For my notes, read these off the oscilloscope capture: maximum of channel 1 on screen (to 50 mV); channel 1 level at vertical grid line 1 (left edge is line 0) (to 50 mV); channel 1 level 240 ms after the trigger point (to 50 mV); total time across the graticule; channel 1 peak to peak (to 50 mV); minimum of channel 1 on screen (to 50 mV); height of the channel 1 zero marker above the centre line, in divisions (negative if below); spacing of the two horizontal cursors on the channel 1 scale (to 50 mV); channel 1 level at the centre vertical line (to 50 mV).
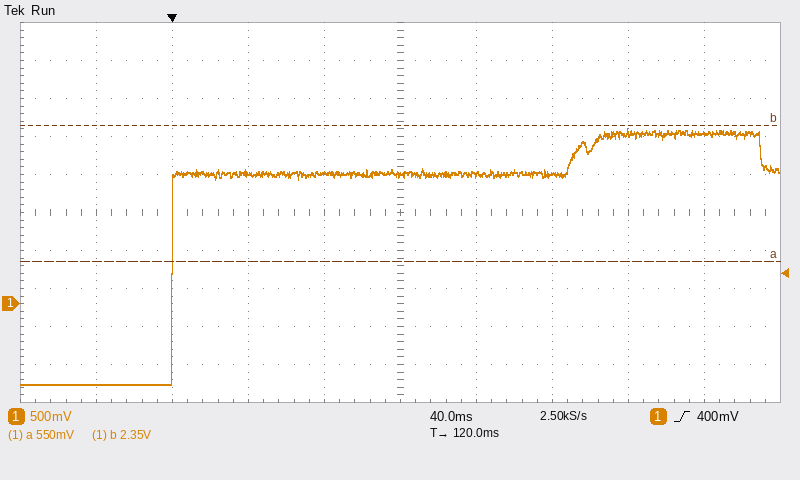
2.30 V
-1.05 V
2.25 V
400 ms
3.35 V
-1.05 V
-2.4 div
1.80 V
1.70 V
